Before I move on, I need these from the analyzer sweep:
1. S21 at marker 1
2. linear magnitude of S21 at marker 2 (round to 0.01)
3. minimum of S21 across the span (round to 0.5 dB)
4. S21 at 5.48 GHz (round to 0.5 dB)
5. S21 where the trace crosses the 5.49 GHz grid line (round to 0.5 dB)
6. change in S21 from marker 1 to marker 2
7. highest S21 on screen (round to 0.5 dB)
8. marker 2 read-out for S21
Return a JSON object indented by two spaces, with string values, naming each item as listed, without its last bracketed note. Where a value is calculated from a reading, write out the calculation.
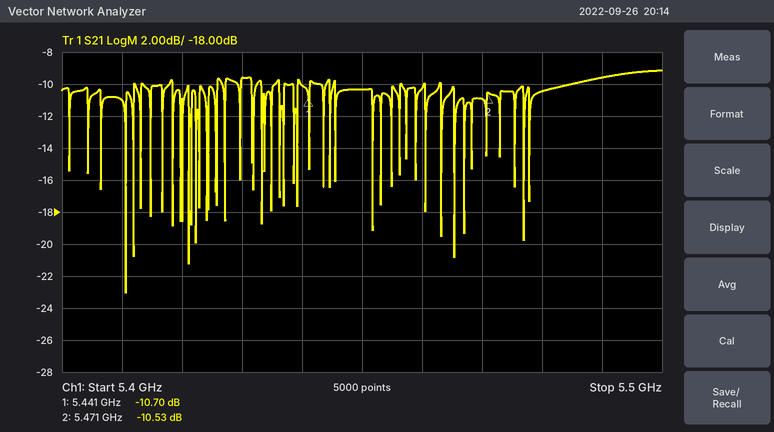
{
  "S21 at marker 1": "-10.70 dB",
  "linear magnitude of S21 at marker 2": "10^(-10.53/20) ≈ 0.30",
  "minimum of S21 across the span": "-23.0 dB",
  "S21 at 5.48 GHz": "-10.5 dB",
  "S21 where the trace crosses the 5.49 GHz grid line": "-9.5 dB",
  "change in S21 from marker 1 to marker 2": "-10.53 − (-10.7) = 0.17 dB",
  "highest S21 on screen": "-9.0 dB",
  "marker 2 read-out for S21": "-10.53 dB"
}
